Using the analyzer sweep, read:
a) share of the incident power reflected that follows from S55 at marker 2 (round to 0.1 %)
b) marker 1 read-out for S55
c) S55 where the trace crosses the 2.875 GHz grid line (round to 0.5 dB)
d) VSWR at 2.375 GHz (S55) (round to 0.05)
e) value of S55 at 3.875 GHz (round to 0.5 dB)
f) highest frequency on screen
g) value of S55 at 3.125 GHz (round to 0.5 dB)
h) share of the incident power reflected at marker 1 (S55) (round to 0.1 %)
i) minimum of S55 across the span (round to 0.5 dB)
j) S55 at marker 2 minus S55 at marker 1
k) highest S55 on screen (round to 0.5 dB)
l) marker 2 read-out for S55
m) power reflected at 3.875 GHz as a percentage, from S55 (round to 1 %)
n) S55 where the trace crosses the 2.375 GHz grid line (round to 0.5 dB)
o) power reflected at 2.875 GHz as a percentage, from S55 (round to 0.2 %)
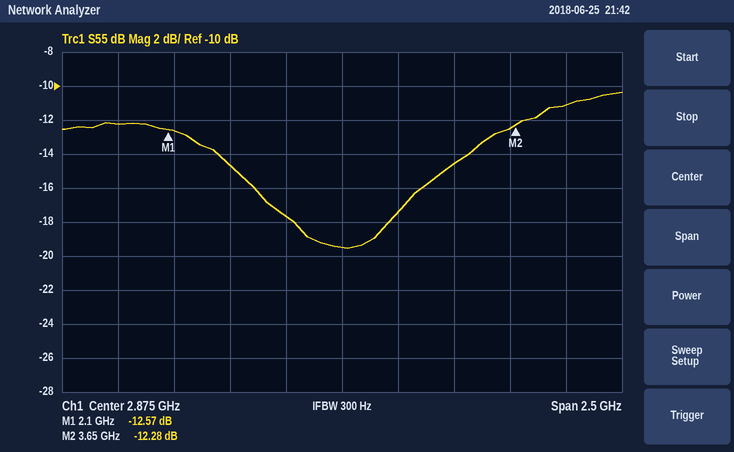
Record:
5.9 %
-12.57 dB
-19.5 dB
1.45
-11.0 dB
4.125 GHz
-17.5 dB
5.5 %
-19.5 dB
0.29 dB
-10.5 dB
-12.28 dB
8 %
-14.5 dB
1.2 %
